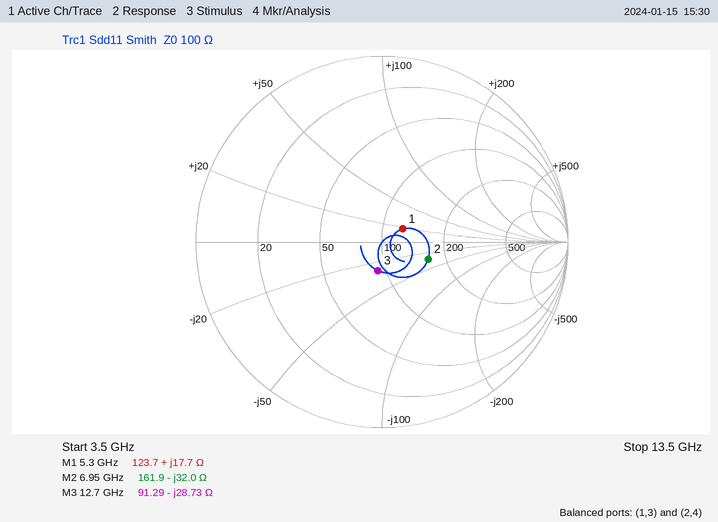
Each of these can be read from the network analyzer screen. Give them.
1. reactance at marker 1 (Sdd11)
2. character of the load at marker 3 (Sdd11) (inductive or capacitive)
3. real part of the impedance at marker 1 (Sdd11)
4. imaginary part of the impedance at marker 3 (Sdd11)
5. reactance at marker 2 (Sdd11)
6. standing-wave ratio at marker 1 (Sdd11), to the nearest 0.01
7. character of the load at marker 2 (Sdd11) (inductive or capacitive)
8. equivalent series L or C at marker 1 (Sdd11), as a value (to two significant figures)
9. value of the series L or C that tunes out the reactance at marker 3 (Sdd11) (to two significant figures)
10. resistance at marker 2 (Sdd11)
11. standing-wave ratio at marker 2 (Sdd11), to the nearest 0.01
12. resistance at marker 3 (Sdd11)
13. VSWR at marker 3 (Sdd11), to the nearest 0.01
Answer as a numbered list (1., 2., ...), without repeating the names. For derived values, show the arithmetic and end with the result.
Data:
1. +17.7 Ω
2. capacitive
3. 123.7 Ω
4. -28.73 Ω
5. -32.0 Ω
6. 1.30
7. capacitive
8. L = 17.7 Ω/(2π × 5.3 GHz) ≈ 532 pH, so 530 pH to two significant figures
9. L = 28.73 Ω/(2π × 12.7 GHz) ≈ 360 pH
10. 161.9 Ω
11. 1.72
12. 91.29 Ω
13. 1.37
